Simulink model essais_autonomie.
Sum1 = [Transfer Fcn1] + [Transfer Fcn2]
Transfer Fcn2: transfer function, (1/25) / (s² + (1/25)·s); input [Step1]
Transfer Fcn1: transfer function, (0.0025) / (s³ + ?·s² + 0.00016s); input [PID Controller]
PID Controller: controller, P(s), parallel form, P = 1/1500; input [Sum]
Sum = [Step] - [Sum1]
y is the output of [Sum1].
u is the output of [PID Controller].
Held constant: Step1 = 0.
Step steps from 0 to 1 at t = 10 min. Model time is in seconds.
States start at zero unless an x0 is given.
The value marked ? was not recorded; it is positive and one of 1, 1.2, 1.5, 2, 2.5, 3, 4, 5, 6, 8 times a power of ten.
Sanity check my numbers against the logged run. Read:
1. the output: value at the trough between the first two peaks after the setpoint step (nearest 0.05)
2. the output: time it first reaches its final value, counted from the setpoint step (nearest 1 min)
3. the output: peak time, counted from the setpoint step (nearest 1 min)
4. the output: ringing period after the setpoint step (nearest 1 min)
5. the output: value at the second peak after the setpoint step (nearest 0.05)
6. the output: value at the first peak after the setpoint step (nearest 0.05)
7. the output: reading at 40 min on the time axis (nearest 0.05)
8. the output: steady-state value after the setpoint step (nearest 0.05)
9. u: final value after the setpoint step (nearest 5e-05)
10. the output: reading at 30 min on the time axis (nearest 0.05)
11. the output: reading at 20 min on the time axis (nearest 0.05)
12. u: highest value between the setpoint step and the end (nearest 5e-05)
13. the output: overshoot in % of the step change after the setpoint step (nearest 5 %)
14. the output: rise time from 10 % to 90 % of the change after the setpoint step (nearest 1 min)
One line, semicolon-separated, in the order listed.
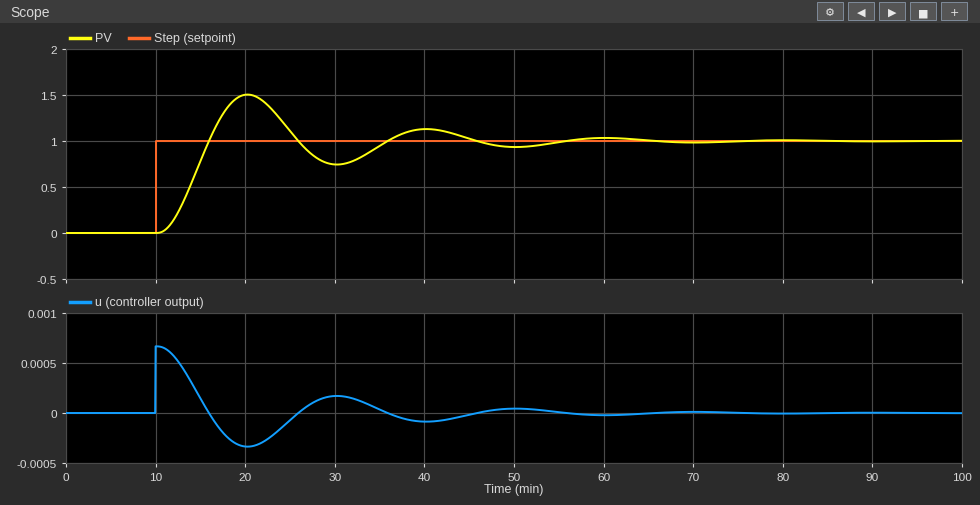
0.75; 6 min; 10 min; 20 min; 1.15; 1.50; 1.15; 1.00; 0.00000; 0.75; 1.50; 0.00065; 50 %; 4 min
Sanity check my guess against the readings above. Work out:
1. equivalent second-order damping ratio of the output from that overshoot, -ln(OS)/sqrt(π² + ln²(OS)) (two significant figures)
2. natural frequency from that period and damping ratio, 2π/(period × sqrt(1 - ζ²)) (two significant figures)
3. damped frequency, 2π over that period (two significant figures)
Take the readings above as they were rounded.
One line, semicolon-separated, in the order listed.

0.22; 0.32 rad/min; 0.31 rad/min
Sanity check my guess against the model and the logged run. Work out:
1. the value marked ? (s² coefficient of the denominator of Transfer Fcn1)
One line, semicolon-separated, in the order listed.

0.06
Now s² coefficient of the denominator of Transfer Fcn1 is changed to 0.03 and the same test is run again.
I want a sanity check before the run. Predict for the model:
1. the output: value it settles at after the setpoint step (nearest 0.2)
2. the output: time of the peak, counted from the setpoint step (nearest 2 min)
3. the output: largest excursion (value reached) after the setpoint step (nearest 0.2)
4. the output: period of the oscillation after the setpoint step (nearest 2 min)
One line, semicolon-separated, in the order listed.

1.0; 8 min; 1.4; 14 min
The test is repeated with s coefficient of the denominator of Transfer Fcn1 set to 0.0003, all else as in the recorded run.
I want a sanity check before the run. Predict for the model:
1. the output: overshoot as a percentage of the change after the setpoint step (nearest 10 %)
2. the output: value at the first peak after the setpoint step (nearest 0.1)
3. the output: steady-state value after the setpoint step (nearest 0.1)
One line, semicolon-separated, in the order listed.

20 %; 1.2; 1.0
